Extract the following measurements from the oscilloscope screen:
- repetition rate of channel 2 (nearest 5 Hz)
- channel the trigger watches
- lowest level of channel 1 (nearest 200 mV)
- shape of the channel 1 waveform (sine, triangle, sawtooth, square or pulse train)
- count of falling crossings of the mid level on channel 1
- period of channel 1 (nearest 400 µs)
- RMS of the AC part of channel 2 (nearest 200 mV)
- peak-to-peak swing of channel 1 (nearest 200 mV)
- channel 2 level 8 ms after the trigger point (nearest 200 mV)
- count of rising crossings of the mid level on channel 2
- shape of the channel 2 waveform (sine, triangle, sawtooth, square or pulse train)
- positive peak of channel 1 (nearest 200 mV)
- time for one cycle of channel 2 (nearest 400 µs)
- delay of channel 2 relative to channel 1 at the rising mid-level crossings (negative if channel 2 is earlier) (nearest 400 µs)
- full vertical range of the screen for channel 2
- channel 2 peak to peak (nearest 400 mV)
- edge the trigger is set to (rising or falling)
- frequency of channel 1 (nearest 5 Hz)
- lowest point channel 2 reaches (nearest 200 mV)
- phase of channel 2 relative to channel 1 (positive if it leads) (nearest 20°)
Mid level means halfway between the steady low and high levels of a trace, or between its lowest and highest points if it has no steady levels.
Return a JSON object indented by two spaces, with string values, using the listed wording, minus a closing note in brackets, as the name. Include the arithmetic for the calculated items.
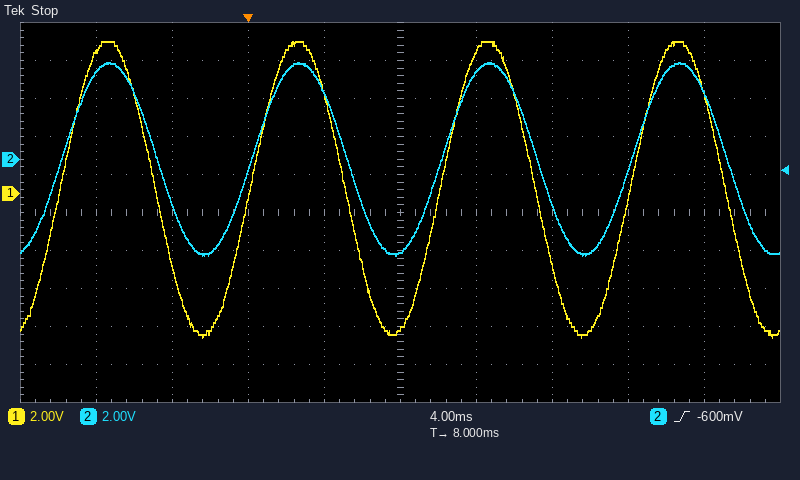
{
  "repetition rate of channel 2": "1 / 10.0 ms ≈ 100 Hz",
  "channel the trigger watches": "channel 2",
  "lowest level of channel 1": "-7.6 V",
  "shape of the channel 1 waveform": "sine",
  "count of falling crossings of the mid level on channel 1": "4",
  "period of channel 1": "10.0 ms",
  "RMS of the AC part of channel 2": "10.0 V / (2√2) ≈ 3.54 V, so 3.6 V to the nearest 200 mV",
  "peak-to-peak swing of channel 1": "8.0 V − (-7.6 V) = 15.6 V",
  "channel 2 level 8 ms after the trigger point": "-4.8 V",
  "count of rising crossings of the mid level on channel 2": "4",
  "shape of the channel 2 waveform": "sine",
  "positive peak of channel 1": "8.0 V",
  "time for one cycle of channel 2": "10.0 ms",
  "delay of channel 2 relative to channel 1 at the rising mid-level crossings (negative if channel 2 is earlier)": "0.0 ms",
  "full vertical range of the screen for channel 2": "20 V",
  "channel 2 peak to peak": "10.0 V",
  "edge the trigger is set to": "rising",
  "frequency of channel 1": "1 / 10.0 ms ≈ 100 Hz",
  "lowest point channel 2 reaches": "-5.0 V",
  "phase of channel 2 relative to channel 1 (positive if it leads)": "−360° × (0.0 ms) / 10.0 ms ≈ 0°"
}
